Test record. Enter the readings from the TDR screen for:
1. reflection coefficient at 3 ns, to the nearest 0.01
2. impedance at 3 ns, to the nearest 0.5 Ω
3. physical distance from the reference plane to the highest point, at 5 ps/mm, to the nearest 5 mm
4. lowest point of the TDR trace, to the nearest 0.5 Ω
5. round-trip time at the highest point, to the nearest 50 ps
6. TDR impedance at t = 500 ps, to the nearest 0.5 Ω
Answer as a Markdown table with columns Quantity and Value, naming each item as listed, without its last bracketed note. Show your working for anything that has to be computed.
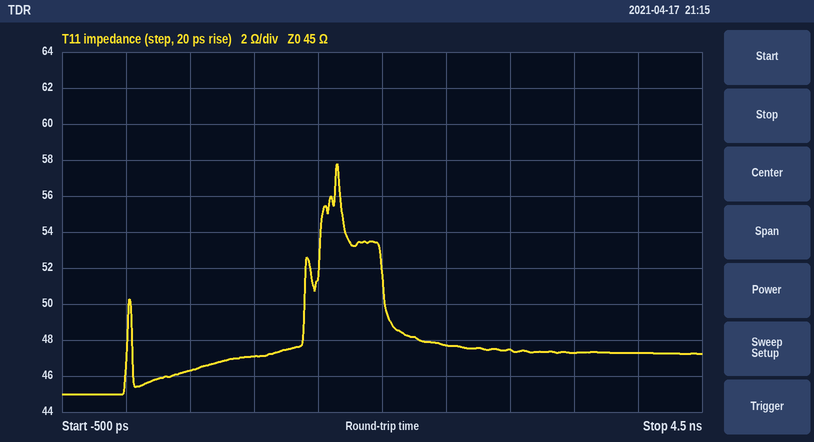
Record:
| Quantity | Value |
|---|---|
| reflection coefficient at 3 ns, to the nearest 0.01 | (47.5 − 45)/(47.5 + 45) ≈ +0.03 |
| impedance at 3 ns, to the nearest 0.5 Ω | 47.5 Ω |
| physical distance from the reference plane to the highest point, at 5 ps/mm, to the nearest 5 mm | 1.65 ns / 2 / 5 ps/mm ≈ 165 mm |
| lowest point of the TDR trace, to the nearest 0.5 Ω | 45.0 Ω |
| round-trip time at the highest point, to the nearest 50 ps | 1.65 ns |
| TDR impedance at t = 500 ps, to the nearest 0.5 Ω | 46.5 Ω |
